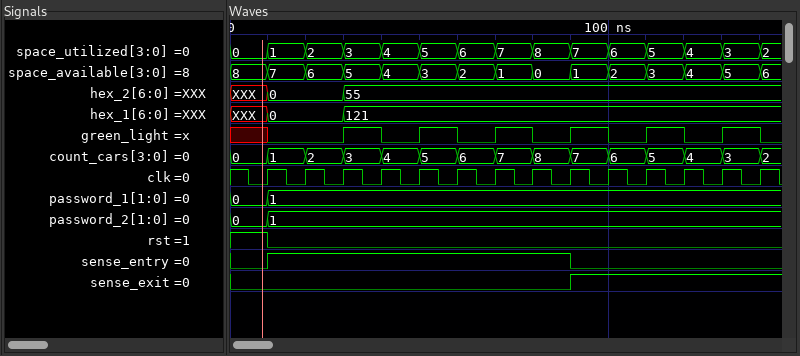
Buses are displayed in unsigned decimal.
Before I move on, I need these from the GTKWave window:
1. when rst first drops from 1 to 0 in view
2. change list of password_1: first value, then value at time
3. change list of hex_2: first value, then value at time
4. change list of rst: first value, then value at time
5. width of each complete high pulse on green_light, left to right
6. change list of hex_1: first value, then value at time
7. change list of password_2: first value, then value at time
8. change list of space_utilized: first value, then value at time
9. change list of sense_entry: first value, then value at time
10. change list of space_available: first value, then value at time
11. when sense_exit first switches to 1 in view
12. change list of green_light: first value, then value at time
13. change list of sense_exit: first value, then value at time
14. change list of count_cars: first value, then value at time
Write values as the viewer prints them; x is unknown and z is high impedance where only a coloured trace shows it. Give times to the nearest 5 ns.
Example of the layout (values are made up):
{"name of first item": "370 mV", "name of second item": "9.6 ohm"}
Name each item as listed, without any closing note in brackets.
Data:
{"when rst first drops from 1 to 0 in view": "10 ns", "change list of password_1: first value, then value at time": "0, 1 at 10 ns", "change list of hex_2: first value, then value at time": "XXX, 0 at 10 ns, 55 at 30 ns", "change list of rst: first value, then value at time": "1, 0 at 10 ns", "width of each complete high pulse on green_light, left to right": "10 ns, 10 ns, 10 ns, 10 ns, 10 ns, 10 ns", "change list of hex_1: first value, then value at time": "XXX, 0 at 10 ns, 121 at 30 ns", "change list of password_2: first value, then value at time": "0, 1 at 10 ns", "change list of space_utilized: first value, then value at time": "0, 1 at 10 ns, 2 at 20 ns, 3 at 30 ns, 4 at 40 ns, 5 at 50 ns, 6 at 60 ns, 7 at 70 ns, 8 at 80 ns, 7 at 90 ns, 6 at 100 ns, 5 at 110 ns, 4 at 120 ns, 3 at 130 ns, 2 at 140 ns", "change list of sense_entry: first value, then value at time": "0, 1 at 10 ns, 0 at 90 ns", "change list of space_available: first value, then value at time": "8, 7 at 10 ns, 6 at 20 ns, 5 at 30 ns, 4 at 40 ns, 3 at 50 ns, 2 at 60 ns, 1 at 70 ns, 0 at 80 ns, 1 at 90 ns, 2 at 100 ns, 3 at 110 ns, 4 at 120 ns, 5 at 130 ns, 6 at 140 ns", "when sense_exit first switches to 1 in view": "90 ns", "change list of green_light: first value, then value at time": "x, 0 at 10 ns, 1 at 30 ns, 0 at 40 ns, 1 at 50 ns, 0 at 60 ns, 1 at 70 ns, 0 at 80 ns, 1 at 90 ns, 0 at 100 ns, 1 at 110 ns, 0 at 120 ns, 1 at 130 ns, 0 at 140 ns", "change list of sense_exit: first value, then value at time": "0, 1 at 90 ns", "change list of count_cars: first value, then value at time": "0, 1 at 10 ns, 2 at 20 ns, 3 at 30 ns, 4 at 40 ns, 5 at 50 ns, 6 at 60 ns, 7 at 70 ns, 8 at 80 ns, 7 at 90 ns, 6 at 100 ns, 5 at 110 ns, 4 at 120 ns, 3 at 130 ns, 2 at 140 ns"}
